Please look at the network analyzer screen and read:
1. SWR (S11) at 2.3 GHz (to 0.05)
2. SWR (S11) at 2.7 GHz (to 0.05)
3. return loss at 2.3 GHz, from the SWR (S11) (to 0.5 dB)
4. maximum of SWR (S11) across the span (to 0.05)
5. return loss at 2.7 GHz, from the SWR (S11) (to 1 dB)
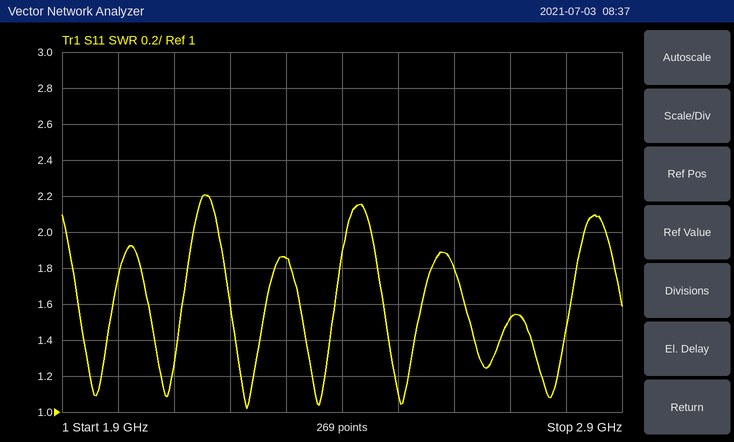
1.85
1.50
10.5 dB
2.20
14 dB
